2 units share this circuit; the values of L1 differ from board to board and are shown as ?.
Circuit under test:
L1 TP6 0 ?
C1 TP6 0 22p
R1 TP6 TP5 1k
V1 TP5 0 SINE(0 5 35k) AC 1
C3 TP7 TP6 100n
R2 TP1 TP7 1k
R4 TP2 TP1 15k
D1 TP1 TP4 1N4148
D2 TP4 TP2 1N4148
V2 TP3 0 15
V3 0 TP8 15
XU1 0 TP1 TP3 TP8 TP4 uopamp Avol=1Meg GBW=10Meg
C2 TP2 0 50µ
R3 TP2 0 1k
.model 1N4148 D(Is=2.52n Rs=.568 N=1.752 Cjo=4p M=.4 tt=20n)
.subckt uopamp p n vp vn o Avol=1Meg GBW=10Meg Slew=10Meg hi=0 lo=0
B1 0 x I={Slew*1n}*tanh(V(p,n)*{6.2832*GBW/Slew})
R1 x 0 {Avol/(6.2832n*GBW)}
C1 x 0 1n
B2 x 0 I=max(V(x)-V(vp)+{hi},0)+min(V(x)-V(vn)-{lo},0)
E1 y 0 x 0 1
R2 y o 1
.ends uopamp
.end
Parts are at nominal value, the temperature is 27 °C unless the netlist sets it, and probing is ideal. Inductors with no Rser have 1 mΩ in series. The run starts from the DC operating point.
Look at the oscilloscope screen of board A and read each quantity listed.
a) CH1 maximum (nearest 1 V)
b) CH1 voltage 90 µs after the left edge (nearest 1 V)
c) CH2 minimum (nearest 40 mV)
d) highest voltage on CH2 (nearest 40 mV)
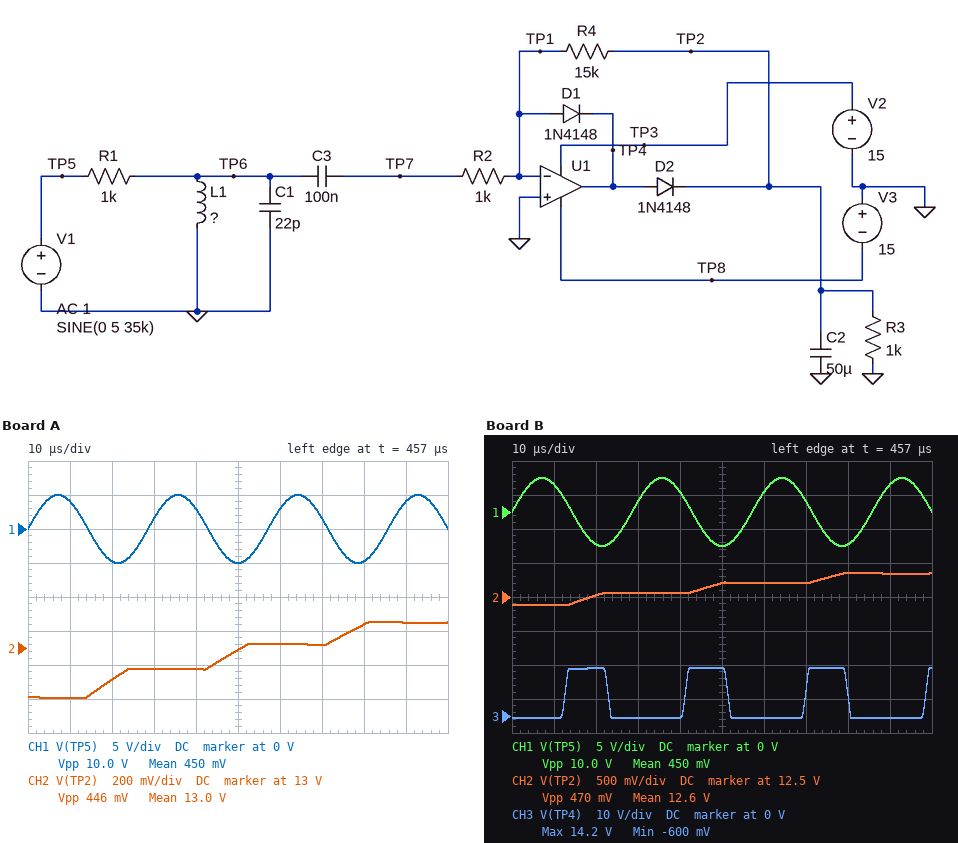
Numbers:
5 V
4 V
12.72 V
13.16 V
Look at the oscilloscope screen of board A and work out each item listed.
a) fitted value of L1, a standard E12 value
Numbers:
3.3 mH
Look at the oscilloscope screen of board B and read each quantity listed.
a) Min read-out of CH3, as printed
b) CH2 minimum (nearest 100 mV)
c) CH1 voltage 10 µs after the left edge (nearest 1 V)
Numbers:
-600 mV
12.4 V
4 V
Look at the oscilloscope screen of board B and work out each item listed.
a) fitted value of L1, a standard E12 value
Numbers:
1.8 mH
